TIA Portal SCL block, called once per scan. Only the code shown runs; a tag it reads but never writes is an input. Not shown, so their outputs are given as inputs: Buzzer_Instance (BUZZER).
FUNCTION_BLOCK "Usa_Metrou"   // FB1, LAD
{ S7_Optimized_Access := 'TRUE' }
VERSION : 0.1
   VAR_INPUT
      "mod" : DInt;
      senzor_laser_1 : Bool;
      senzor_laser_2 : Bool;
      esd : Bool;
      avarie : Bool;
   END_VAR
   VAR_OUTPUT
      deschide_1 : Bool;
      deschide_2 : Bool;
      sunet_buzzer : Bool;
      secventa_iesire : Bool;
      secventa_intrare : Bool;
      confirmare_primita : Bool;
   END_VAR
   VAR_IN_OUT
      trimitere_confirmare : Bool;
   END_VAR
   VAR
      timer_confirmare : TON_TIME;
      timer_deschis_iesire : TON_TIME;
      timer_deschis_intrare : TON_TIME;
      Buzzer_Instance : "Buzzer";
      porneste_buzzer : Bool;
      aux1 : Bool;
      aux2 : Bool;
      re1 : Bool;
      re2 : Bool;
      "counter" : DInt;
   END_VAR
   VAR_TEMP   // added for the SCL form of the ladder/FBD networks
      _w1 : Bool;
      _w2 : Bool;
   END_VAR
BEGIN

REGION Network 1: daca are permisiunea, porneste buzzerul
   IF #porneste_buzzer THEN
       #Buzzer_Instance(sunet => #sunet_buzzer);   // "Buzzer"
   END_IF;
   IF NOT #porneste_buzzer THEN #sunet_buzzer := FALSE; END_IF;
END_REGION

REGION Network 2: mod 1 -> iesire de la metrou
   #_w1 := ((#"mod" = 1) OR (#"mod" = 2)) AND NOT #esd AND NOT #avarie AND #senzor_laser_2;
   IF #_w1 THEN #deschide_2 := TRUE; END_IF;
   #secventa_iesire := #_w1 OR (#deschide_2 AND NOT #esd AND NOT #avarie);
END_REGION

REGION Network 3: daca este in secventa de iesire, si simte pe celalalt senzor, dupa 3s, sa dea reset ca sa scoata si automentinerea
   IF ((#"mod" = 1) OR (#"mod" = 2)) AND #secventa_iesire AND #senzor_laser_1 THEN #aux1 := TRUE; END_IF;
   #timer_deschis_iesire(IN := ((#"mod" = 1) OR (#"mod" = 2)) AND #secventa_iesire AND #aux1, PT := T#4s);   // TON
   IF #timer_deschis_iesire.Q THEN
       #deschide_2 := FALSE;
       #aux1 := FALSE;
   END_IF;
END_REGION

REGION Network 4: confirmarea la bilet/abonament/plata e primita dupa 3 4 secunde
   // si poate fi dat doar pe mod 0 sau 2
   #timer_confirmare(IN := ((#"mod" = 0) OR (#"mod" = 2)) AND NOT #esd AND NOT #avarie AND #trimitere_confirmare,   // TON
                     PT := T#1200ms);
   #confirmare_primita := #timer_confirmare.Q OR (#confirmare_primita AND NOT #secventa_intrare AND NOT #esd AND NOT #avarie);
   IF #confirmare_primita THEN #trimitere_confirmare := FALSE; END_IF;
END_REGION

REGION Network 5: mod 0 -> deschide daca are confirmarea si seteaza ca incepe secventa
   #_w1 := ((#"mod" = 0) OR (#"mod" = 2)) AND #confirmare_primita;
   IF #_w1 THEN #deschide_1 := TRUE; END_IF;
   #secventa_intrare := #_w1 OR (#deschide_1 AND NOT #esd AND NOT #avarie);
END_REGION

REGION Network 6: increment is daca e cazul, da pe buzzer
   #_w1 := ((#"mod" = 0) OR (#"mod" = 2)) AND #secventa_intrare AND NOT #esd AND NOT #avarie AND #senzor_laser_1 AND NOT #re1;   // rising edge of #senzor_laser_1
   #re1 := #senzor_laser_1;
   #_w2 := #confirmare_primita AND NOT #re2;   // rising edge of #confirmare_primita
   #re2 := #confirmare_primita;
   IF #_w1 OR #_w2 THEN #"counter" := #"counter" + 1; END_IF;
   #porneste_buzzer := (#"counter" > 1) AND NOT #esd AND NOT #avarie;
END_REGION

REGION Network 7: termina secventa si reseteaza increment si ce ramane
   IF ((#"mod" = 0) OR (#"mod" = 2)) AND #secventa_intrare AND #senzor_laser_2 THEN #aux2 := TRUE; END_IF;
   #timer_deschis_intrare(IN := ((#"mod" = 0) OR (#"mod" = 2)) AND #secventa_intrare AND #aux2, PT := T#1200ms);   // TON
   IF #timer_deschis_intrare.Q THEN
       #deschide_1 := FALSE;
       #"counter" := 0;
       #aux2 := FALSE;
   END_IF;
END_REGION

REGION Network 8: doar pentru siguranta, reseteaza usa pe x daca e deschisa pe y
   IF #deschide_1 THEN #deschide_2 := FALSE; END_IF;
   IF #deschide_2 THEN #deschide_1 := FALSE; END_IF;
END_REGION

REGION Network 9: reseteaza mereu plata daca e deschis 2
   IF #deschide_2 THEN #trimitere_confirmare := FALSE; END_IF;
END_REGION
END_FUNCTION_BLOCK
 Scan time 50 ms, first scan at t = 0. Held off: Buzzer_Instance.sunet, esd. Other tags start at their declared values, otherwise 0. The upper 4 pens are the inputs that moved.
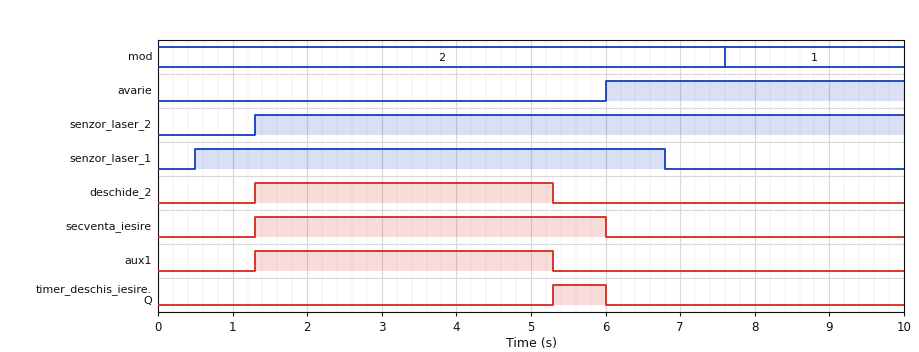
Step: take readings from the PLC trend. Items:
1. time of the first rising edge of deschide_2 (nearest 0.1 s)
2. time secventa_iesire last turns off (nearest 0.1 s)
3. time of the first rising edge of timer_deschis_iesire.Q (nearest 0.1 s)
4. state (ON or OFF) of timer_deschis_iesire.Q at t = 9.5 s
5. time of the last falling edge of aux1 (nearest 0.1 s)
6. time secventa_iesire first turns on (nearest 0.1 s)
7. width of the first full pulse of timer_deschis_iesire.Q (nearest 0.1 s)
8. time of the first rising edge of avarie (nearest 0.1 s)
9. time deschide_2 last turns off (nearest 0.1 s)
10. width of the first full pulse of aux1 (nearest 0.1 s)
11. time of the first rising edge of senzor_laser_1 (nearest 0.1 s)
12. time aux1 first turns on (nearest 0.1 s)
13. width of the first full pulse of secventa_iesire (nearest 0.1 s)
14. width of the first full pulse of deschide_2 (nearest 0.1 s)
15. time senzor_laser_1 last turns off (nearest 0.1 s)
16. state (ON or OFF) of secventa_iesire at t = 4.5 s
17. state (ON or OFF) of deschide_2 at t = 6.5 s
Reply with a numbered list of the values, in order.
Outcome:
1. 1.3 s
2. 6.0 s
3. 5.3 s
4. OFF
5. 5.3 s
6. 1.3 s
7. 0.7 s
8. 6.0 s
9. 5.3 s
10. 4.0 s
11. 0.5 s
12. 1.3 s
13. 4.7 s
14. 4.0 s
15. 6.8 s
16. ON
17. OFF
